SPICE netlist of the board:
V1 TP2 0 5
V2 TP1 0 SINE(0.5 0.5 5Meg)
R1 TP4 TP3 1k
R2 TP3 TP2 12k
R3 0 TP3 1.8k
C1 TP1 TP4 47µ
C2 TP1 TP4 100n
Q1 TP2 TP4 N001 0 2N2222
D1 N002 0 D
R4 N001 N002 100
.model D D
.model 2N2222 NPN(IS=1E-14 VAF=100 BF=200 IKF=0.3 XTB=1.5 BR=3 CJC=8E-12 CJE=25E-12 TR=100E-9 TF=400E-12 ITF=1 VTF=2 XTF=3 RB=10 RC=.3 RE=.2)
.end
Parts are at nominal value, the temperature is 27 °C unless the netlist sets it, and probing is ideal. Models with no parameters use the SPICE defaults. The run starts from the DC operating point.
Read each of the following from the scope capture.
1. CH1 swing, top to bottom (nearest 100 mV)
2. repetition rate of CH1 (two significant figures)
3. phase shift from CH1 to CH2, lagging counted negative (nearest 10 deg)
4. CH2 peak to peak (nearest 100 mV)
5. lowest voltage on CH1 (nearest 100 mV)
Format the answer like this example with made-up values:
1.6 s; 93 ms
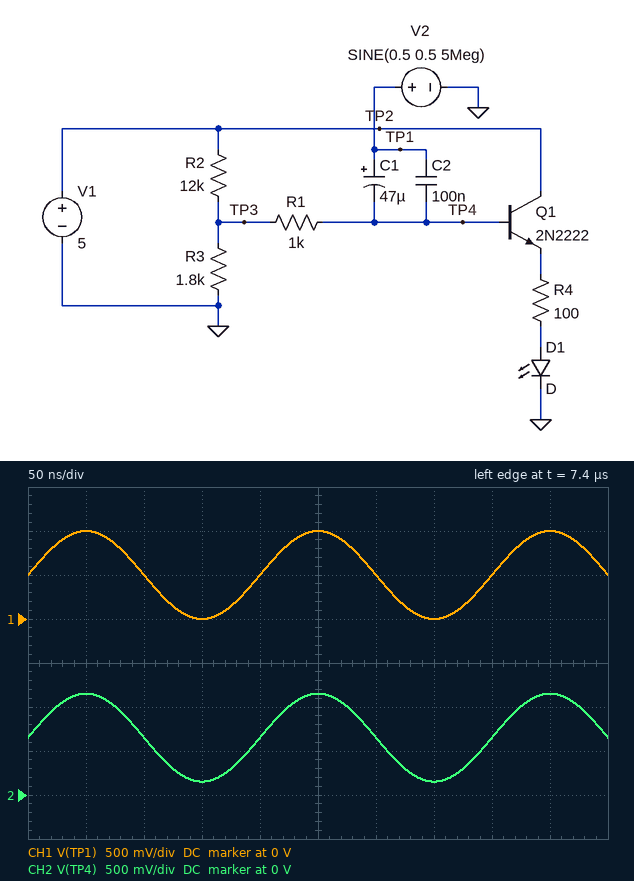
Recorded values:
1.0 V; 5.0 MHz; 0 deg; 1.0 V; 0 V
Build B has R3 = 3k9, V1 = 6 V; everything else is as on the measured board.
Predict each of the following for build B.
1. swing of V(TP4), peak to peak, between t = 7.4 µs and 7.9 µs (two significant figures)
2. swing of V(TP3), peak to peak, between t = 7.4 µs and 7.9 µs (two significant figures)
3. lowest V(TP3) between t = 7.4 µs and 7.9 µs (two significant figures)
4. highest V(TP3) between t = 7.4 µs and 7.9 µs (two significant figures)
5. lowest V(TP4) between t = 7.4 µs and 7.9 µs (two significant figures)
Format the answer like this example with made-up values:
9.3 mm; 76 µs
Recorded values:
1.0 V; 750 mV; 1.1 V; 1.8 V; 950 mV
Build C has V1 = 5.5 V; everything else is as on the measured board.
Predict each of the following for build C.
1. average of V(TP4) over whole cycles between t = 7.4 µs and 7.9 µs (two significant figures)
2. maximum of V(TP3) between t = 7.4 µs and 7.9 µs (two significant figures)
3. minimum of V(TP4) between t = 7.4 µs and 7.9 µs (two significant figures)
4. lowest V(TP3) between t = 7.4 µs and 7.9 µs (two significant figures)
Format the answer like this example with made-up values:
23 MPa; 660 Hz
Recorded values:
720 mV; 1.0 V; 220 mV; 410 mV
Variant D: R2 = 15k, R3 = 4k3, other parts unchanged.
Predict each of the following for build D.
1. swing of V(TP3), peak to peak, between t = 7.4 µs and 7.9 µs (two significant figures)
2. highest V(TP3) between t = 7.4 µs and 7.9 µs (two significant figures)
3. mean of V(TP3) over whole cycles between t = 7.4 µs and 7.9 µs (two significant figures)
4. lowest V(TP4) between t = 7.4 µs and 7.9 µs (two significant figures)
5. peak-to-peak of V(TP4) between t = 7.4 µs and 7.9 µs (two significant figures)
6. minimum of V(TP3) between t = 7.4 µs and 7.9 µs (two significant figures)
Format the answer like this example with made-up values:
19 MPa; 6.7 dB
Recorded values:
770 mV; 1.5 V; 1.1 V; 610 mV; 1.0 V; 730 mV
